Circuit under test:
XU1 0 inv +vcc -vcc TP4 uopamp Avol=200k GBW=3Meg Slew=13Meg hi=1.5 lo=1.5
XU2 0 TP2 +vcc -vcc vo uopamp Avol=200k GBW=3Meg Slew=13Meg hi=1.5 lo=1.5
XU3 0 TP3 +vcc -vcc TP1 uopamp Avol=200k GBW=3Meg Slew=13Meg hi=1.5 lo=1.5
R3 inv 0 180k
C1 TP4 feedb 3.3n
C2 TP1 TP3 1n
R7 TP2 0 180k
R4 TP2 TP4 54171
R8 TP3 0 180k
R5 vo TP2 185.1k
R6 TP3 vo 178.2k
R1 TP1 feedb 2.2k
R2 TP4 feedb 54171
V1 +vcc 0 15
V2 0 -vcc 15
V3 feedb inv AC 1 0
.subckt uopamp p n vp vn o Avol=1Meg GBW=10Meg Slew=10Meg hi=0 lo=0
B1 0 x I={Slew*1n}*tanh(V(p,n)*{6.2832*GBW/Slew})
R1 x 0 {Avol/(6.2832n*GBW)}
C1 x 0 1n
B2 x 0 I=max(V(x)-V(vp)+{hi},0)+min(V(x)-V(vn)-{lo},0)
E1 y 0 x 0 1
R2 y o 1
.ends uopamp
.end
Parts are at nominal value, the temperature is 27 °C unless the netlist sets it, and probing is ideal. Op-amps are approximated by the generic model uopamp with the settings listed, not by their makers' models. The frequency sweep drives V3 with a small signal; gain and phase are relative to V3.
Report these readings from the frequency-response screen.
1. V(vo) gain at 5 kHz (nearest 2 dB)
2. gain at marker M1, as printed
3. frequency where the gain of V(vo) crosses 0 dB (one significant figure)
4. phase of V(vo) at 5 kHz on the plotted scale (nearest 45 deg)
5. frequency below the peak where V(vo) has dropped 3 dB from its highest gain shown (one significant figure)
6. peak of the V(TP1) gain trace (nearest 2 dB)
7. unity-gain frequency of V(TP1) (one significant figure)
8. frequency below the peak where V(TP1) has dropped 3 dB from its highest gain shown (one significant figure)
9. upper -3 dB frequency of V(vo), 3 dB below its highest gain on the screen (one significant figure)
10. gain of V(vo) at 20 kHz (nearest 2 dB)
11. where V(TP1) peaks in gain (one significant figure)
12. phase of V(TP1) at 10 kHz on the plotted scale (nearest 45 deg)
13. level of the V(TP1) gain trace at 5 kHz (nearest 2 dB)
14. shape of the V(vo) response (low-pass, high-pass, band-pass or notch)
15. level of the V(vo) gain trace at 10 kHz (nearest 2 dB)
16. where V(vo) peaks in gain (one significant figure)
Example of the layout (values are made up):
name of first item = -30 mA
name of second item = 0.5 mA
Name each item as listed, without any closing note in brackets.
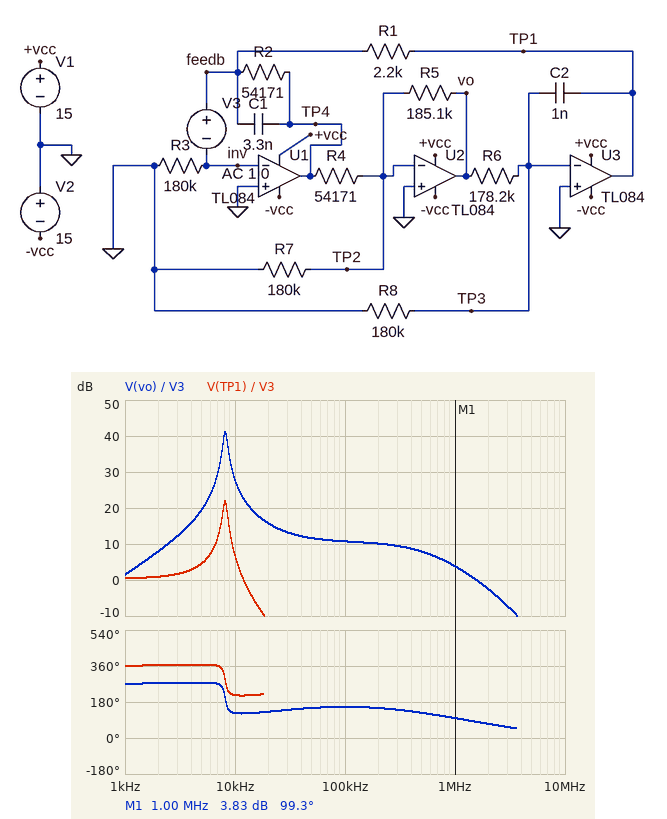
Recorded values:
V(vo) gain at 5 kHz = 20 dB
gain at marker M1, as printed = 3.83 dB
frequency where the gain of V(vo) crosses 0 dB = 2 MHz
phase of V(vo) at 5 kHz on the plotted scale = 270 deg
frequency below the peak where V(vo) has dropped 3 dB from its highest gain shown = 8 kHz
peak of the V(TP1) gain trace = 22 dB
unity-gain frequency of V(TP1) = 10 kHz
frequency below the peak where V(TP1) has dropped 3 dB from its highest gain shown = 8 kHz
upper -3 dB frequency of V(vo), 3 dB below its highest gain on the screen = 9 kHz
gain of V(vo) at 20 kHz = 16 dB
where V(TP1) peaks in gain = 8 kHz
phase of V(TP1) at 10 kHz on the plotted scale = 225 deg
level of the V(TP1) gain trace at 5 kHz = 4 dB
shape of the V(vo) response = band-pass
level of the V(vo) gain trace at 10 kHz = 28 dB
where V(vo) peaks in gain = 8 kHz
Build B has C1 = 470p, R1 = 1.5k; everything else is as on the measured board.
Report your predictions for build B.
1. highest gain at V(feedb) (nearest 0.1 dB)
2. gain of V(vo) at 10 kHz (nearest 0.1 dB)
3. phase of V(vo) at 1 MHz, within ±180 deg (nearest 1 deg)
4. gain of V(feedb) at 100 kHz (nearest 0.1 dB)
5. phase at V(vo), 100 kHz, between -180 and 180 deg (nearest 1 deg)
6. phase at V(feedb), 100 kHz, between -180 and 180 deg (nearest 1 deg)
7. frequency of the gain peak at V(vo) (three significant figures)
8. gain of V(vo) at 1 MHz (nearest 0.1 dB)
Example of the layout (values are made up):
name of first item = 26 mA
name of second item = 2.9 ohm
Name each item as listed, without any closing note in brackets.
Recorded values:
highest gain at V(feedb) = 1.9 dB
gain of V(vo) at 10 kHz = 22.7 dB
phase of V(vo) at 1 MHz, within ±180 deg = 89 deg
gain of V(feedb) at 100 kHz = -0.7 dB
phase at V(vo), 100 kHz, between -180 and 180 deg = 104 deg
phase at V(feedb), 100 kHz, between -180 and 180 deg = -2 deg
frequency of the gain peak at V(vo) = 25.3 kHz
gain of V(vo) at 1 MHz = 3.5 dB
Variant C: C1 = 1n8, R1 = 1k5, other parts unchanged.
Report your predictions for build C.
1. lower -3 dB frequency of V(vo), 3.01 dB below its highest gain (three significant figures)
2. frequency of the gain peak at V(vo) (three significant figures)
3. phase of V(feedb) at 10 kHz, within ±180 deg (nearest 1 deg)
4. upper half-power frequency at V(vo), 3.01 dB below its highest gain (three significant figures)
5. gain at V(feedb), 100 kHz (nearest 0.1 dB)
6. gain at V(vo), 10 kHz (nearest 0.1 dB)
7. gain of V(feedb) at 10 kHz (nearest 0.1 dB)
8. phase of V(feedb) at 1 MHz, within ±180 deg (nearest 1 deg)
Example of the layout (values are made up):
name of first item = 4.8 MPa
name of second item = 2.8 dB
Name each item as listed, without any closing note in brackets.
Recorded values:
lower -3 dB frequency of V(vo), 3.01 dB below its highest gain = 12.7 kHz
frequency of the gain peak at V(vo) = 13.3 kHz
phase of V(feedb) at 10 kHz, within ±180 deg = 0 deg
upper half-power frequency at V(vo), 3.01 dB below its highest gain = 13.9 kHz
gain at V(feedb), 100 kHz = -0.2 dB
gain at V(vo), 10 kHz = 28.5 dB
gain of V(feedb) at 10 kHz = 0.2 dB
phase of V(feedb) at 1 MHz, within ±180 deg = -18 deg
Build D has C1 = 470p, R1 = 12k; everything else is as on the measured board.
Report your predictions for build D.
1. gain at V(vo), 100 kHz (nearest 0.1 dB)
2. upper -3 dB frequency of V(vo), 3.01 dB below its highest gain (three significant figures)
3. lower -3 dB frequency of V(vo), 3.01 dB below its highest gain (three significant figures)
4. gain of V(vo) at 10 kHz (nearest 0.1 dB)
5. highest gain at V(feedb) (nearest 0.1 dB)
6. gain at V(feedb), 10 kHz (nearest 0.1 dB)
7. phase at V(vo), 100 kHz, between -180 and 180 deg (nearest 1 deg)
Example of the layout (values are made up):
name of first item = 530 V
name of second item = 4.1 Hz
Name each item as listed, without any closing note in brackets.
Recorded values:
gain at V(vo), 100 kHz = 11.0 dB
upper -3 dB frequency of V(vo), 3.01 dB below its highest gain = 12.9 kHz
lower -3 dB frequency of V(vo), 3.01 dB below its highest gain = 6.78 kHz
gain of V(vo) at 10 kHz = 25.9 dB
highest gain at V(feedb) = 0.1 dB
gain at V(feedb), 10 kHz = 0 dB
phase at V(vo), 100 kHz, between -180 and 180 deg = 152 deg
